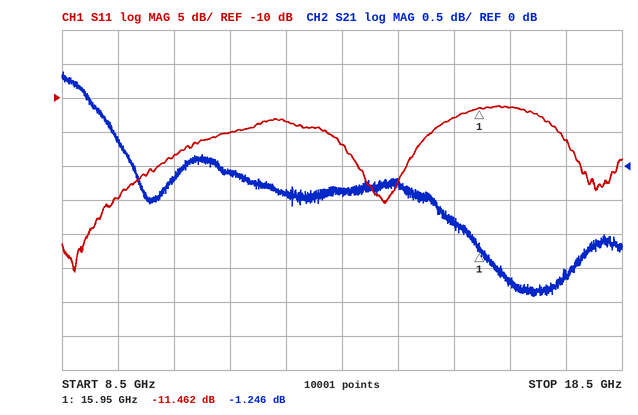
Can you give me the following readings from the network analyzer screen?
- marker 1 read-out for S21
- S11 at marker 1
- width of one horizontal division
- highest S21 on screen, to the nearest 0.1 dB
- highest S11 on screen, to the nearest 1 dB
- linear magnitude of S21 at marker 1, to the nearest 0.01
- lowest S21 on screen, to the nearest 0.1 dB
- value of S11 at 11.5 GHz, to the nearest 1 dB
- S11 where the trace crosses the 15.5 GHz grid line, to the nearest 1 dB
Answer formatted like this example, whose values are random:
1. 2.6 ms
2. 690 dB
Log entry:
1. -1.246 dB
2. -11.462 dB
3. 1 GHz
4. 1.4 dB
5. -11 dB
6. 0.87
7. -1.9 dB
8. -15 dB
9. -13 dB
